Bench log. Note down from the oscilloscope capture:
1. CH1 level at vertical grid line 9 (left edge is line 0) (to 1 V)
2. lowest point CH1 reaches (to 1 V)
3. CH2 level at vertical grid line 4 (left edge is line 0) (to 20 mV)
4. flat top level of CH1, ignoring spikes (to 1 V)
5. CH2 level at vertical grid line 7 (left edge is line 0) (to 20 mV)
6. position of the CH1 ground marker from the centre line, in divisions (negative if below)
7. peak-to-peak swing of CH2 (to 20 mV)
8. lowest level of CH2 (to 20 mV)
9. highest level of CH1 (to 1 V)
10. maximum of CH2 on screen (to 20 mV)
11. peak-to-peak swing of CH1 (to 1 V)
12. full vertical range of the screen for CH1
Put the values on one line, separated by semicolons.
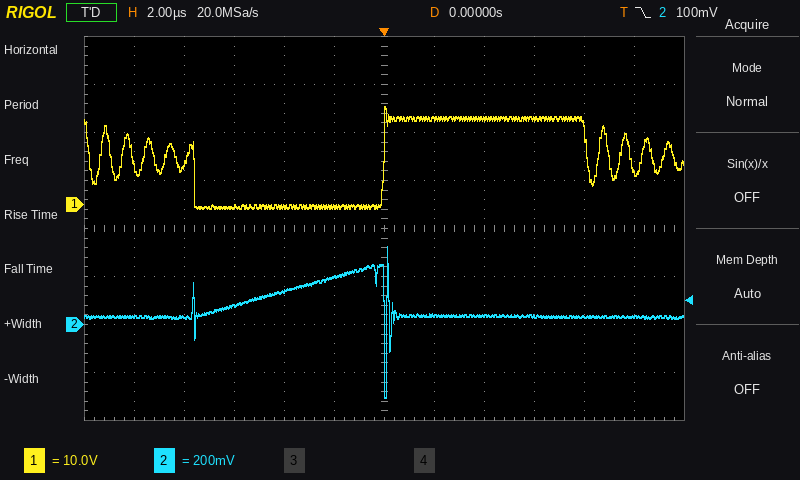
18 V; -1 V; 140 mV; 18 V; 40 mV; +0.5 div; 620 mV; -300 mV; 20 V; 320 mV; 21 V; 80 V
